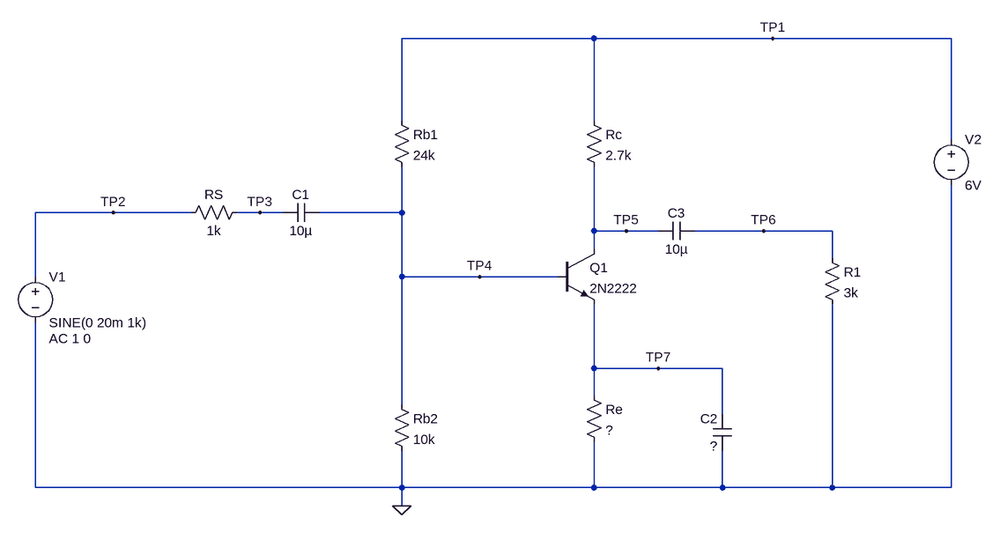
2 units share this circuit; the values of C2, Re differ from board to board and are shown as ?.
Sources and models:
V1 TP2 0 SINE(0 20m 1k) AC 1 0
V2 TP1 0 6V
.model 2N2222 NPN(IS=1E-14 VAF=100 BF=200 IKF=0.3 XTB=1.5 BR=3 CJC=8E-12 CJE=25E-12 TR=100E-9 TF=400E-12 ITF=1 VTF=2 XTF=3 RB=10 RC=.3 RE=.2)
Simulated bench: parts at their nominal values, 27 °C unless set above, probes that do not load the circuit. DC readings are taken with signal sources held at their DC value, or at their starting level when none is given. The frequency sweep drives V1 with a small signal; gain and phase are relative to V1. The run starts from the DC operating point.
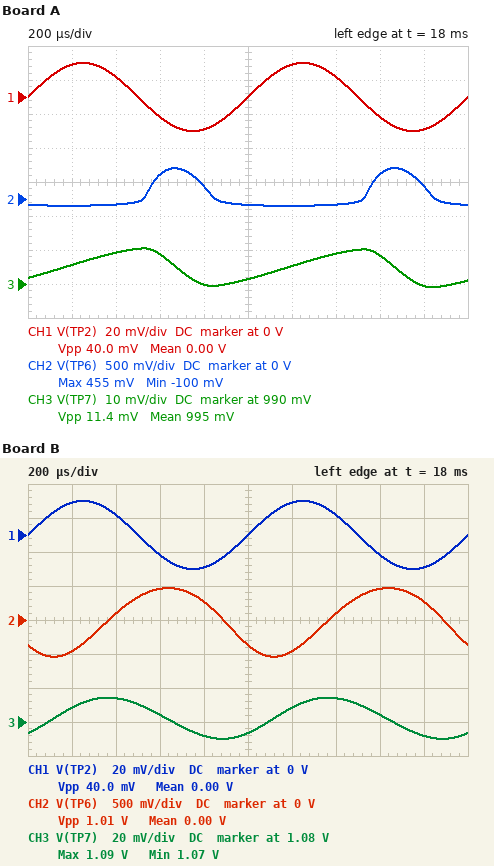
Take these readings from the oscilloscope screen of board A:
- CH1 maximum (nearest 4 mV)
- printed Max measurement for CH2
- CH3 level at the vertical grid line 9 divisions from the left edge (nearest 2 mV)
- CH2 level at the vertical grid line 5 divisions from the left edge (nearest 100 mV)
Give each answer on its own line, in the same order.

20 mV
455 mV
990 mV
-100 mV
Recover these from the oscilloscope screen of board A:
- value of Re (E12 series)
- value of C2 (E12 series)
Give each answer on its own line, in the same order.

560 Ω
5.6 µF
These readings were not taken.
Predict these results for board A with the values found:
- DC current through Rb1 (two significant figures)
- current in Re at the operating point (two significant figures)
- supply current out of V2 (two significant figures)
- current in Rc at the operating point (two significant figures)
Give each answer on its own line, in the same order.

180 µA
1.8 mA
2.0 mA
1.8 mA
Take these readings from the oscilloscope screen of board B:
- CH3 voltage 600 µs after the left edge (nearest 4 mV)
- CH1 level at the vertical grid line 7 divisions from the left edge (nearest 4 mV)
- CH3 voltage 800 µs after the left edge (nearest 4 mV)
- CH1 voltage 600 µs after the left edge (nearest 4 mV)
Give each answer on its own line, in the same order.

1.084 V
12 mV
1.072 V
-12 mV
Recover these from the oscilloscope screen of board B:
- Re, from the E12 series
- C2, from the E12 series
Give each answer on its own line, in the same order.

1.2 kΩ
4.7 µF
